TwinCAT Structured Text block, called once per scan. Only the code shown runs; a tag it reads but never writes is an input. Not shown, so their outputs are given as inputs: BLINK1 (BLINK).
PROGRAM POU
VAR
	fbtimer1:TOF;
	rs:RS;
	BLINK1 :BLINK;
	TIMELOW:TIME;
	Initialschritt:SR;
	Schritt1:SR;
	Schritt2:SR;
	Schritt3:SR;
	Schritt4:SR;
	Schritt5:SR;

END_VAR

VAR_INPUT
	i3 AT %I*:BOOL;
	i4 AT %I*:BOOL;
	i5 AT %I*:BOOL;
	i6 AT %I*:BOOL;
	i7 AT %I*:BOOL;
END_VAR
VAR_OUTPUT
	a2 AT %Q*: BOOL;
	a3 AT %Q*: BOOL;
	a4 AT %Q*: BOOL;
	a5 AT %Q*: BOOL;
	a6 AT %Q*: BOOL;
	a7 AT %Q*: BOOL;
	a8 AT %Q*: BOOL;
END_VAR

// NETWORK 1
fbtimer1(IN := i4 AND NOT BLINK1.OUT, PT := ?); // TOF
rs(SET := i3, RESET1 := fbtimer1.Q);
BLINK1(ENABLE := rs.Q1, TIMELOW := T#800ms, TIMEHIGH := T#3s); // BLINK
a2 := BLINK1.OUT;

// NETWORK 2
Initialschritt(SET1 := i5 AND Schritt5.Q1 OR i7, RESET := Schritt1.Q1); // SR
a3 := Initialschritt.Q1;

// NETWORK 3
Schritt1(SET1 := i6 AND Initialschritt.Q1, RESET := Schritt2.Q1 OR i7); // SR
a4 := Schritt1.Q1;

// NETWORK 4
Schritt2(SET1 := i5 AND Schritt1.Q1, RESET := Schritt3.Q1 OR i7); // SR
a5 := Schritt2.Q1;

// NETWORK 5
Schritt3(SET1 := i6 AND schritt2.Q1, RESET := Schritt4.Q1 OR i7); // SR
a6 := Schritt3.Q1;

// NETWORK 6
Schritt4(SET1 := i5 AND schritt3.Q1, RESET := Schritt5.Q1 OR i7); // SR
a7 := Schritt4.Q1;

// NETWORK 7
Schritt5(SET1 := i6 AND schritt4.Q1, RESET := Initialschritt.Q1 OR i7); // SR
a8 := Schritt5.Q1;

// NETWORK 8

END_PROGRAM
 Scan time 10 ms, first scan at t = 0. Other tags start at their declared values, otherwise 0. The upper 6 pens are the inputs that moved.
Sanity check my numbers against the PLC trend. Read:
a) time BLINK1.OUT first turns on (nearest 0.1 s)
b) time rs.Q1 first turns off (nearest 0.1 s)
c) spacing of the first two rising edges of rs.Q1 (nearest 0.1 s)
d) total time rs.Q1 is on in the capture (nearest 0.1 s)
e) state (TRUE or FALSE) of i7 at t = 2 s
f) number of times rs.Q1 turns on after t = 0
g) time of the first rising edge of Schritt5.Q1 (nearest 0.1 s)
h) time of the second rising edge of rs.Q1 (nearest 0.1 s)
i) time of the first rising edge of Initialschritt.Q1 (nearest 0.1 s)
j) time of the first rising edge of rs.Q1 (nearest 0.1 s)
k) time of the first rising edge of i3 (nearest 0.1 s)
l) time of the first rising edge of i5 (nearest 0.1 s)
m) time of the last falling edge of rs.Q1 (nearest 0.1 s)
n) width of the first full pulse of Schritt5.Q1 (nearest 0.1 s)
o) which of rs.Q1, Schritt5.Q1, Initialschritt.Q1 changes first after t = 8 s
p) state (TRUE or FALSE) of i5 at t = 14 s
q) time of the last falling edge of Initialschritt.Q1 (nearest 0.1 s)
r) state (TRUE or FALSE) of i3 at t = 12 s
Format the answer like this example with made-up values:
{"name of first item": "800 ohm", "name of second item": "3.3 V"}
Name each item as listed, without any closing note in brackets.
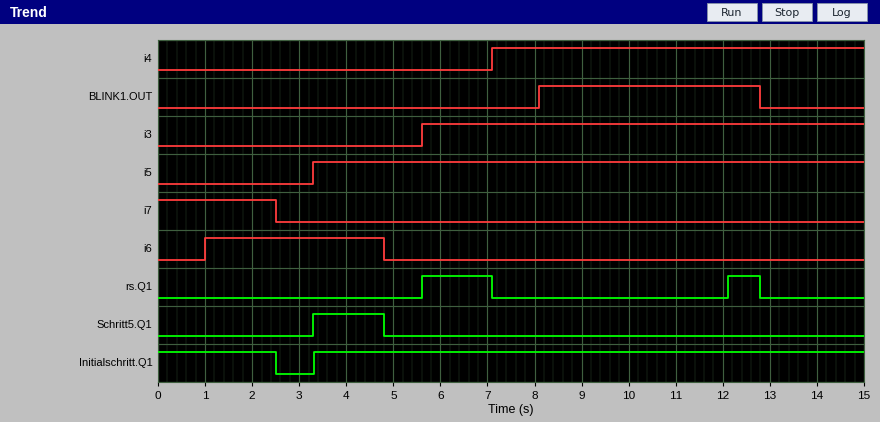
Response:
{"time BLINK1.OUT first turns on": "8.1 s", "time rs.Q1 first turns off": "7.1 s", "spacing of the first two rising edges of rs.Q1": "6.5 s", "total time rs.Q1 is on in the capture": "2.2 s", "state (TRUE or FALSE) of i7 at t = 2 s": "TRUE", "number of times rs.Q1 turns on after t = 0": "2", "time of the first rising edge of Schritt5.Q1": "3.3 s", "time of the second rising edge of rs.Q1": "12.1 s", "time of the first rising edge of Initialschritt.Q1": "3.3 s", "time of the first rising edge of rs.Q1": "5.6 s", "time of the first rising edge of i3": "5.6 s", "time of the first rising edge of i5": "3.3 s", "time of the last falling edge of rs.Q1": "12.8 s", "width of the first full pulse of Schritt5.Q1": "1.5 s", "which of rs.Q1, Schritt5.Q1, Initialschritt.Q1 changes first after t = 8 s": "rs.Q1", "state (TRUE or FALSE) of i5 at t = 14 s": "TRUE", "time of the last falling edge of Initialschritt.Q1": "2.5 s", "state (TRUE or FALSE) of i3 at t = 12 s": "TRUE"}
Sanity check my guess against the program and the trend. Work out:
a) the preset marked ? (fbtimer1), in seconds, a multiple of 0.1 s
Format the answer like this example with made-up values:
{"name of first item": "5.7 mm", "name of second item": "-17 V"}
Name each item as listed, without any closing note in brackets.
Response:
{"the preset marked ? (fbtimer1), in seconds, a multiple of 0.1 s": "4.0 s"}
